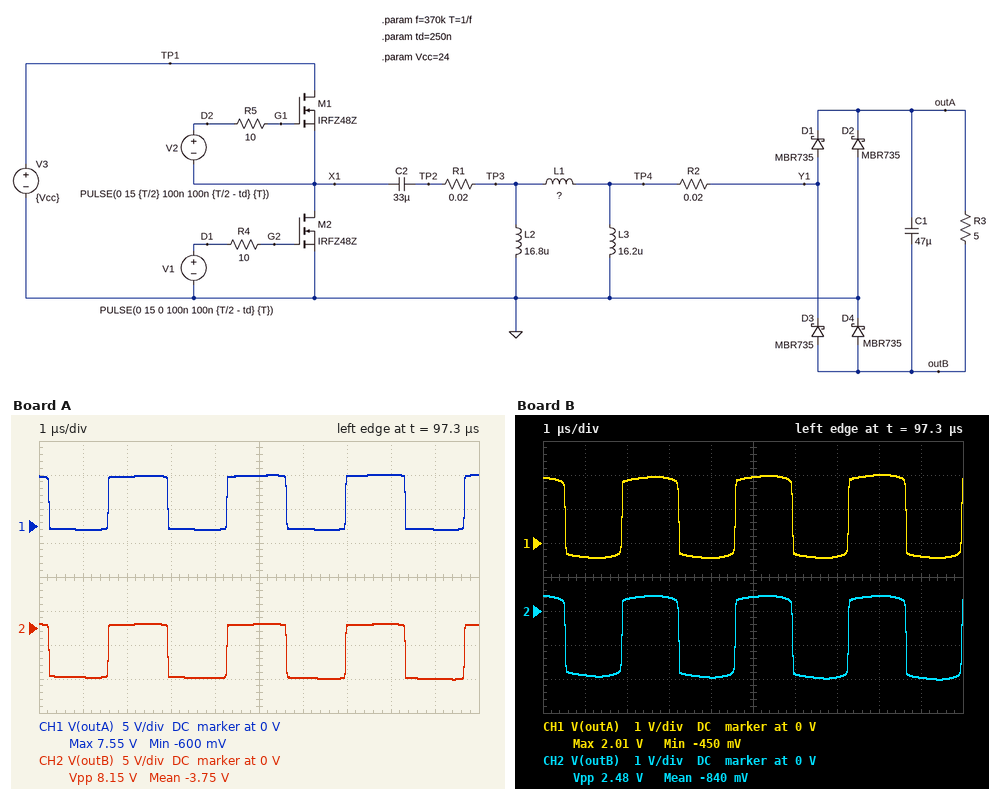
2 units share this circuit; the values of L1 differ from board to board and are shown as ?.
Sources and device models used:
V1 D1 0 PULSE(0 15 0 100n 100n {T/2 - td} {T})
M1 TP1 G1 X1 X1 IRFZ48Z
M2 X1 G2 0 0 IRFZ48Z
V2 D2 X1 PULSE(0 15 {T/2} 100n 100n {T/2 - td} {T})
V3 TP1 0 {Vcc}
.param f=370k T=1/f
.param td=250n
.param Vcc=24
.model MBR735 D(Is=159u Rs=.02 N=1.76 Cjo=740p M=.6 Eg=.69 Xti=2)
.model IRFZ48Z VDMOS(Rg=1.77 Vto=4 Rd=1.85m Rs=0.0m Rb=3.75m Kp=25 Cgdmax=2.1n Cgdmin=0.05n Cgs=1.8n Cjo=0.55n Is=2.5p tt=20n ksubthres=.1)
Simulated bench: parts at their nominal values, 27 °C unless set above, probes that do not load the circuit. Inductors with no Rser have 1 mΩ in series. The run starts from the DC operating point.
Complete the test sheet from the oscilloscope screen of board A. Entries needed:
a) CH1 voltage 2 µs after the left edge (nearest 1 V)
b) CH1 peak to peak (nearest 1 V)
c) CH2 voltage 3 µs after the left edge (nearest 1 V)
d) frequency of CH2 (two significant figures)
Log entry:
7 V
8 V
-7 V
370 kHz
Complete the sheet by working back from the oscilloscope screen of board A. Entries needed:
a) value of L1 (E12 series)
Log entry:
820 nH
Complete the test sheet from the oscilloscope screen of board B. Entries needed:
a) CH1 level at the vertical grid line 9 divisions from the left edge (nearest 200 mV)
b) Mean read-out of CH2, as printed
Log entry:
-400 mV
-840 mV
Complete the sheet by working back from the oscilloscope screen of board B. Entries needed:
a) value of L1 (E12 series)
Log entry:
4.7 µH
